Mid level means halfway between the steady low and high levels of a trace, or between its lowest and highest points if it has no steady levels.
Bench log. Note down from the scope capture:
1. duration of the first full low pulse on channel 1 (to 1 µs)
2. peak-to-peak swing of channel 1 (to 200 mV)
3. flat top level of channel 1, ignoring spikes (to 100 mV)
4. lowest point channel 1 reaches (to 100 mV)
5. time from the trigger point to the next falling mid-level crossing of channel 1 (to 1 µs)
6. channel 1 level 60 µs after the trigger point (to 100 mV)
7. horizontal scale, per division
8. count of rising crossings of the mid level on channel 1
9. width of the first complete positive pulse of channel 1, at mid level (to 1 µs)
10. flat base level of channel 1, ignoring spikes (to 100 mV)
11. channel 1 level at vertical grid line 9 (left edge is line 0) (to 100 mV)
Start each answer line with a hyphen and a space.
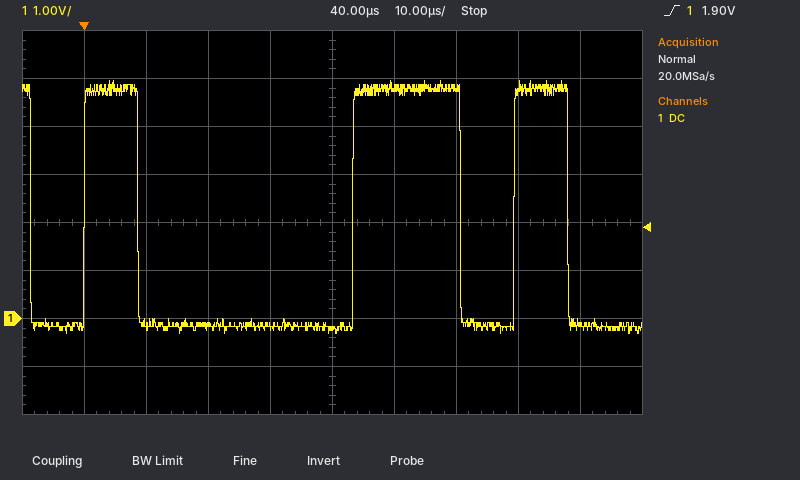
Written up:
- 9 µs
- 5.2 V
- 4.8 V
- -300 mV
- 9 µs
- 4.8 V
- 10 µs
- 3
- 9 µs
- -200 mV
- -100 mV
